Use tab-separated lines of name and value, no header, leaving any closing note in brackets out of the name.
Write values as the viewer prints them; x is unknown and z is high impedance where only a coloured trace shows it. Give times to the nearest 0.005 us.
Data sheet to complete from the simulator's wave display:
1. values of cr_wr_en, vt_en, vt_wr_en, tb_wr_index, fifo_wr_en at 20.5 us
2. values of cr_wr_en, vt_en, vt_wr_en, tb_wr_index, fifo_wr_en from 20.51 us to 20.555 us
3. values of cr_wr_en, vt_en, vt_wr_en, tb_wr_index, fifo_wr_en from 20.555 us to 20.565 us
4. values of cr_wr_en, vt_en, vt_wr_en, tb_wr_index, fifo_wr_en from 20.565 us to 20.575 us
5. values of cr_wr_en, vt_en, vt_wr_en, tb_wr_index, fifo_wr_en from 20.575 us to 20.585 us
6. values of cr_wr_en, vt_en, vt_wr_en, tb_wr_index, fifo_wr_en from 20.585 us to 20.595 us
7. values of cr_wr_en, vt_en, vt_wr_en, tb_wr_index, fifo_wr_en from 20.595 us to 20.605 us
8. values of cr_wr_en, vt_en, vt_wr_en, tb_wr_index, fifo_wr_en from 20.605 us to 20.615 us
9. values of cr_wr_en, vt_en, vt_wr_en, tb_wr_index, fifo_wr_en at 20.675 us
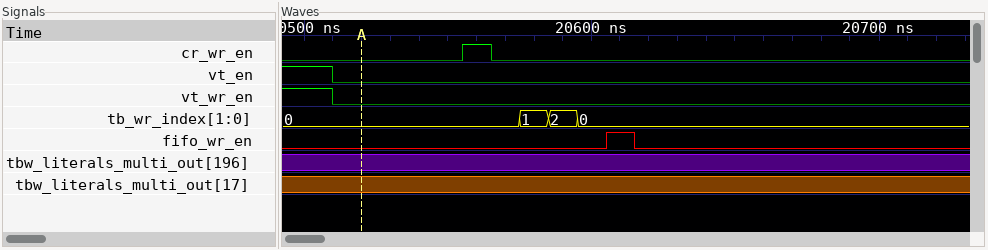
values of cr_wr_en, vt_en, vt_wr_en, tb_wr_index, fifo_wr_en at 20.5 us	cr_wr_en=0, vt_en=1, vt_wr_en=1, tb_wr_index=0, fifo_wr_en=0
values of cr_wr_en, vt_en, vt_wr_en, tb_wr_index, fifo_wr_en from 20.51 us to 20.555 us	cr_wr_en=0, vt_en=0, vt_wr_en=0, tb_wr_index=0, fifo_wr_en=0
values of cr_wr_en, vt_en, vt_wr_en, tb_wr_index, fifo_wr_en from 20.555 us to 20.565 us	cr_wr_en=1, vt_en=0, vt_wr_en=0, tb_wr_index=0, fifo_wr_en=0
values of cr_wr_en, vt_en, vt_wr_en, tb_wr_index, fifo_wr_en from 20.565 us to 20.575 us	cr_wr_en=0, vt_en=0, vt_wr_en=0, tb_wr_index=0, fifo_wr_en=0
values of cr_wr_en, vt_en, vt_wr_en, tb_wr_index, fifo_wr_en from 20.575 us to 20.585 us	cr_wr_en=0, vt_en=0, vt_wr_en=0, tb_wr_index=1, fifo_wr_en=0
values of cr_wr_en, vt_en, vt_wr_en, tb_wr_index, fifo_wr_en from 20.585 us to 20.595 us	cr_wr_en=0, vt_en=0, vt_wr_en=0, tb_wr_index=2, fifo_wr_en=0
values of cr_wr_en, vt_en, vt_wr_en, tb_wr_index, fifo_wr_en from 20.595 us to 20.605 us	cr_wr_en=0, vt_en=0, vt_wr_en=0, tb_wr_index=0, fifo_wr_en=0
values of cr_wr_en, vt_en, vt_wr_en, tb_wr_index, fifo_wr_en from 20.605 us to 20.615 us	cr_wr_en=0, vt_en=0, vt_wr_en=0, tb_wr_index=0, fifo_wr_en=1
values of cr_wr_en, vt_en, vt_wr_en, tb_wr_index, fifo_wr_en at 20.675 us	cr_wr_en=0, vt_en=0, vt_wr_en=0, tb_wr_index=0, fifo_wr_en=0
